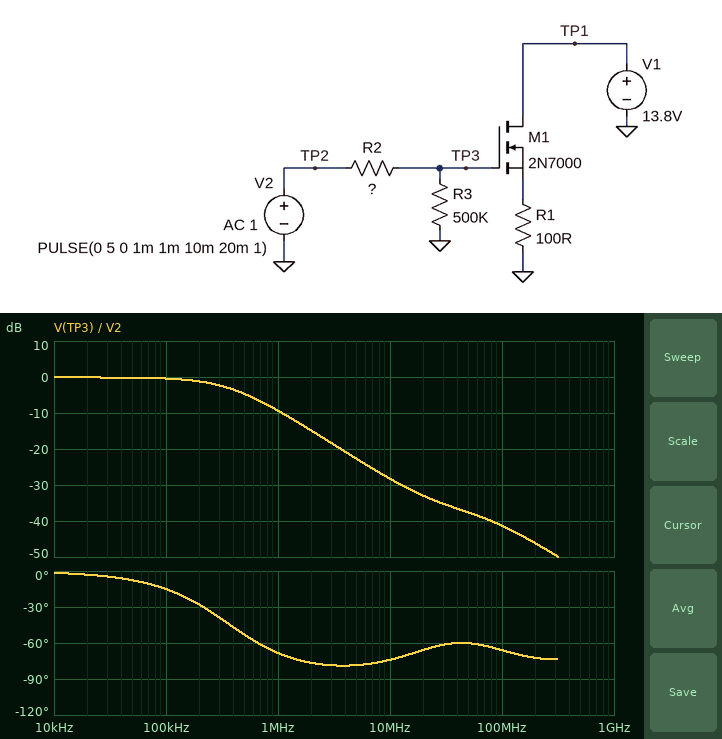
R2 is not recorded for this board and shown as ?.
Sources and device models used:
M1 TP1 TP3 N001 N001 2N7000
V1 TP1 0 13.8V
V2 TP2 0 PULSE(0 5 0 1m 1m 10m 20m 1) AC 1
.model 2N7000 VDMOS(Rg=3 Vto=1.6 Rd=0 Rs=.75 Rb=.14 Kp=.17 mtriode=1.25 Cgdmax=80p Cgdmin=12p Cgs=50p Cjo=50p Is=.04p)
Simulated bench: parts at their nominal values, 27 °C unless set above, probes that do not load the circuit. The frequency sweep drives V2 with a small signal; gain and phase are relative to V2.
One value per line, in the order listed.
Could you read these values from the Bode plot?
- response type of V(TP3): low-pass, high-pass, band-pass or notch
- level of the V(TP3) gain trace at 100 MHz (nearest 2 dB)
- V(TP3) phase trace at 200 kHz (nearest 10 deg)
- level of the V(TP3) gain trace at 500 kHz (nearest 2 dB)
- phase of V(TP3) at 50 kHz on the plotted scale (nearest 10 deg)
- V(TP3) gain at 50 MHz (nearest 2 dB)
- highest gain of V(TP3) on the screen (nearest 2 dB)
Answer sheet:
low-pass
-42 dB
-30 deg
-4 dB
-10 deg
-38 dB
0 dB
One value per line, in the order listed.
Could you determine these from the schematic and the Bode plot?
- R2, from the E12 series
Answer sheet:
6.8 kΩ
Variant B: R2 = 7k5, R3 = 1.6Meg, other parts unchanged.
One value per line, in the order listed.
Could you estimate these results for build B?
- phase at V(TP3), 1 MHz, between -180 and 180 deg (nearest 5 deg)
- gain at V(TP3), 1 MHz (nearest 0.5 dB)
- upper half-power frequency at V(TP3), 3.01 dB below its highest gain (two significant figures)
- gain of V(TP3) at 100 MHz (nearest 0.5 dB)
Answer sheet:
-70 deg
-10.0 dB
330 kHz
-42.0 dB
